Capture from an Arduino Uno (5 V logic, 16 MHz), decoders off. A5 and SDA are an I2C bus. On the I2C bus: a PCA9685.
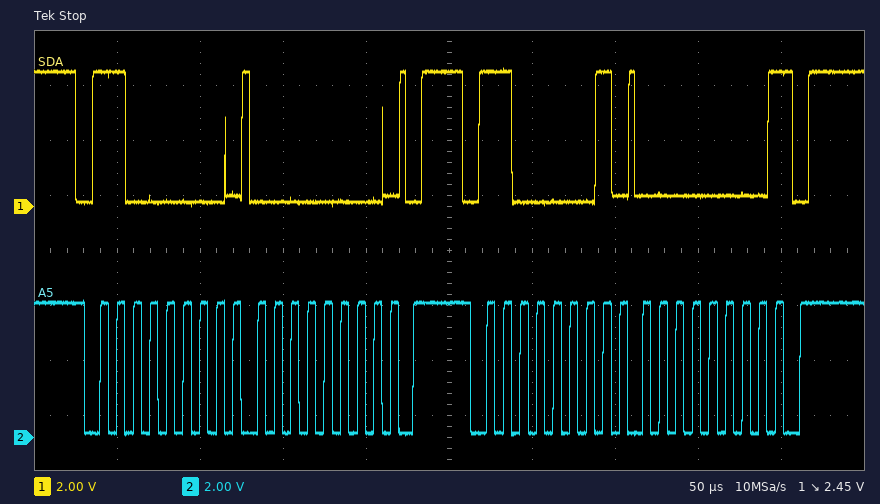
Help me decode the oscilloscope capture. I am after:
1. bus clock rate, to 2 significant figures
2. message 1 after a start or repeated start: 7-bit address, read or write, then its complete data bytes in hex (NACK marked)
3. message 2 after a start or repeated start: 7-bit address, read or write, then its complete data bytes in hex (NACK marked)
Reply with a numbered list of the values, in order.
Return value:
1. 100 kHz
2. 0x60 write: 00
3. 0x60 read: 00 NACK
